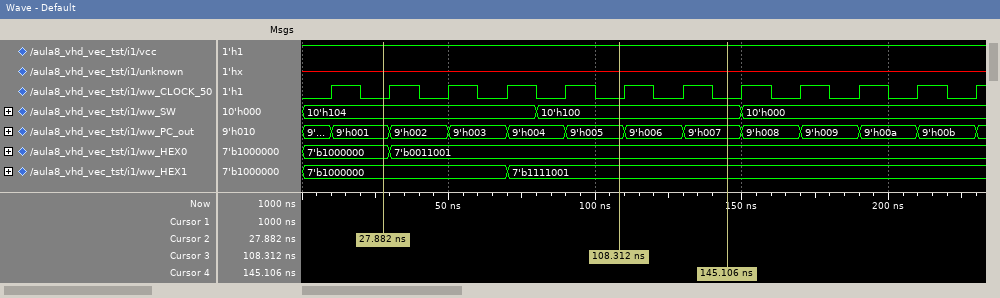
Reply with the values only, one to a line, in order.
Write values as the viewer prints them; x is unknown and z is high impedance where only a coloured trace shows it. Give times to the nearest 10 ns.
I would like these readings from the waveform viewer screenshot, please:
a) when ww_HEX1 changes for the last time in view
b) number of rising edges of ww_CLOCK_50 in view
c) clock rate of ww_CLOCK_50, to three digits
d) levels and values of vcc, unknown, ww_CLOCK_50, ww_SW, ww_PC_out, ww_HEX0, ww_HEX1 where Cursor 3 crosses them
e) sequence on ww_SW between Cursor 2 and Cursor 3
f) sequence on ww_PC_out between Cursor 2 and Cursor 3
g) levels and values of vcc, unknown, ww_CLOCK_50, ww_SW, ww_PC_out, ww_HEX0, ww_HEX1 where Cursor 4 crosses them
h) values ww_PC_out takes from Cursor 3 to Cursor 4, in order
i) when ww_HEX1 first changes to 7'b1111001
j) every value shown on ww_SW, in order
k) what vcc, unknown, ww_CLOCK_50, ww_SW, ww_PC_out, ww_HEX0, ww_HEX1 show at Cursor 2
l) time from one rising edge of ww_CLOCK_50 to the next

70 ns
12
50.0 MHz
vcc=1, unknown=x, ww_CLOCK_50=0, ww_SW=10'h100, ww_PC_out=9'h005, ww_HEX0=7'b0011001, ww_HEX1=7'b1111001
10'h104, 10'h100
9'h001, 9'h002, 9'h003, 9'h004, 9'h005
vcc=1, unknown=x, ww_CLOCK_50=0, ww_SW=10'h100, ww_PC_out=9'h007, ww_HEX0=7'b0011001, ww_HEX1=7'b1111001
9'h005, 9'h006, 9'h007
70 ns
10'h104, 10'h100, 10'h000
vcc=1, unknown=x, ww_CLOCK_50=0, ww_SW=10'h104, ww_PC_out=9'h001, ww_HEX0=7'b1000000, ww_HEX1=7'b1000000
20 ns
